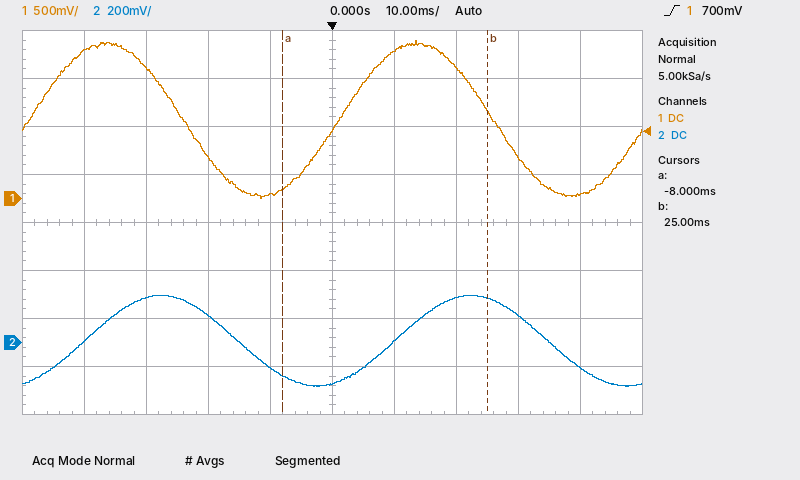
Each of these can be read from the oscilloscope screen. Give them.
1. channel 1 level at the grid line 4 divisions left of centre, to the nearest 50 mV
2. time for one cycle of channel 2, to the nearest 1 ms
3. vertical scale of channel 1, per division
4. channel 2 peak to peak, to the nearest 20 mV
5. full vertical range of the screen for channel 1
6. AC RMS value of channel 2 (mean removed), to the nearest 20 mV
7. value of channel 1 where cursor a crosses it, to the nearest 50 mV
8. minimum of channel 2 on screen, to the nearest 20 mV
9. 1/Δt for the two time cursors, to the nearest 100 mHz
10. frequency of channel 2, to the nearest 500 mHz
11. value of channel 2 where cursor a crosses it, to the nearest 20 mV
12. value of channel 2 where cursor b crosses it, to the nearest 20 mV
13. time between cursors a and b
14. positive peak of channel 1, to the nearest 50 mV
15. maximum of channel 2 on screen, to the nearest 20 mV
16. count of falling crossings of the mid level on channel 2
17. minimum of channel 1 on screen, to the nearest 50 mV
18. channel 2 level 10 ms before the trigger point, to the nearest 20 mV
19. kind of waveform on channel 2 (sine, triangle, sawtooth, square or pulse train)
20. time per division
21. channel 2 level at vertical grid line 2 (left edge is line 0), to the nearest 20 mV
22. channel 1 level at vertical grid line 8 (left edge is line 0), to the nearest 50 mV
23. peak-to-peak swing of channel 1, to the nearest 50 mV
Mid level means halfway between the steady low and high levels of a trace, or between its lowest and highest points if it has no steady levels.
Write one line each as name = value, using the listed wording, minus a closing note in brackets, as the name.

channel 1 level at the grid line 4 divisions left of centre, to the nearest 50 mV = 1.55 V
time for one cycle of channel 2, to the nearest 1 ms = 50 ms
vertical scale of channel 1, per division = 500 mV
channel 2 peak to peak, to the nearest 20 mV = 380 mV
full vertical range of the screen for channel 1 = 4 V
AC RMS value of channel 2 (mean removed), to the nearest 20 mV = 140 mV
value of channel 1 where cursor a crosses it, to the nearest 50 mV = 100 mV
minimum of channel 2 on screen, to the nearest 20 mV = -180 mV
1/Δt for the two time cursors, to the nearest 100 mHz = 30.3 Hz
frequency of channel 2, to the nearest 500 mHz = 20.0 Hz
value of channel 2 where cursor a crosses it, to the nearest 20 mV = -140 mV
value of channel 2 where cursor b crosses it, to the nearest 20 mV = 180 mV
time between cursors a and b = 33 ms
positive peak of channel 1, to the nearest 50 mV = 1.65 V
maximum of channel 2 on screen, to the nearest 20 mV = 200 mV
count of falling crossings of the mid level on channel 2 = 2
minimum of channel 1 on screen, to the nearest 50 mV = 0 mV
channel 2 level 10 ms before the trigger point, to the nearest 20 mV = -100 mV
kind of waveform on channel 2 = sine
time per division = 10 ms
channel 2 level at vertical grid line 2 (left edge is line 0), to the nearest 20 mV = 180 mV
channel 1 level at vertical grid line 8 (left edge is line 0), to the nearest 50 mV = 450 mV
peak-to-peak swing of channel 1, to the nearest 50 mV = 1.65 V
